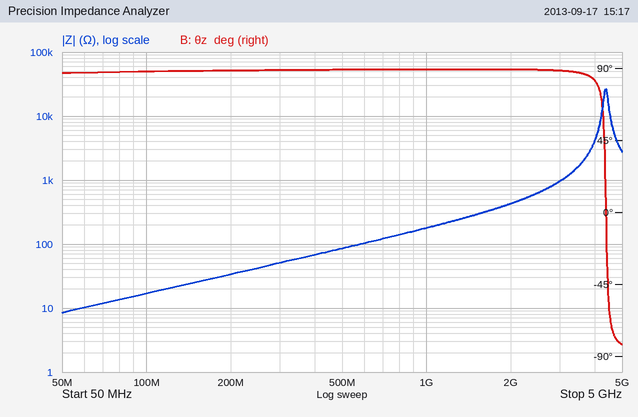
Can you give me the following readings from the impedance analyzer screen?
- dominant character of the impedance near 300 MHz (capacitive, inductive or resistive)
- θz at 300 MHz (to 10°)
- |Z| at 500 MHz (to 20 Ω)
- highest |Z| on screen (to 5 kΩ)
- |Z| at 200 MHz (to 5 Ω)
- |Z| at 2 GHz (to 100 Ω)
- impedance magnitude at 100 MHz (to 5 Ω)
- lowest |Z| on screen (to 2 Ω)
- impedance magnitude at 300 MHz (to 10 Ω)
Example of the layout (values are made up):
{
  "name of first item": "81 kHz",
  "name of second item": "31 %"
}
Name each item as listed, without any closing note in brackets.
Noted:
{
  "dominant character of the impedance near 300 MHz": "inductive",
  "θz at 300 MHz": "90°",
  "|Z| at 500 MHz": "80 Ω",
  "highest |Z| on screen": "25 kΩ",
  "|Z| at 200 MHz": "35 Ω",
  "|Z| at 2 GHz": "400 Ω",
  "impedance magnitude at 100 MHz": "15 Ω",
  "lowest |Z| on screen": "8 Ω",
  "impedance magnitude at 300 MHz": "50 Ω"
}
